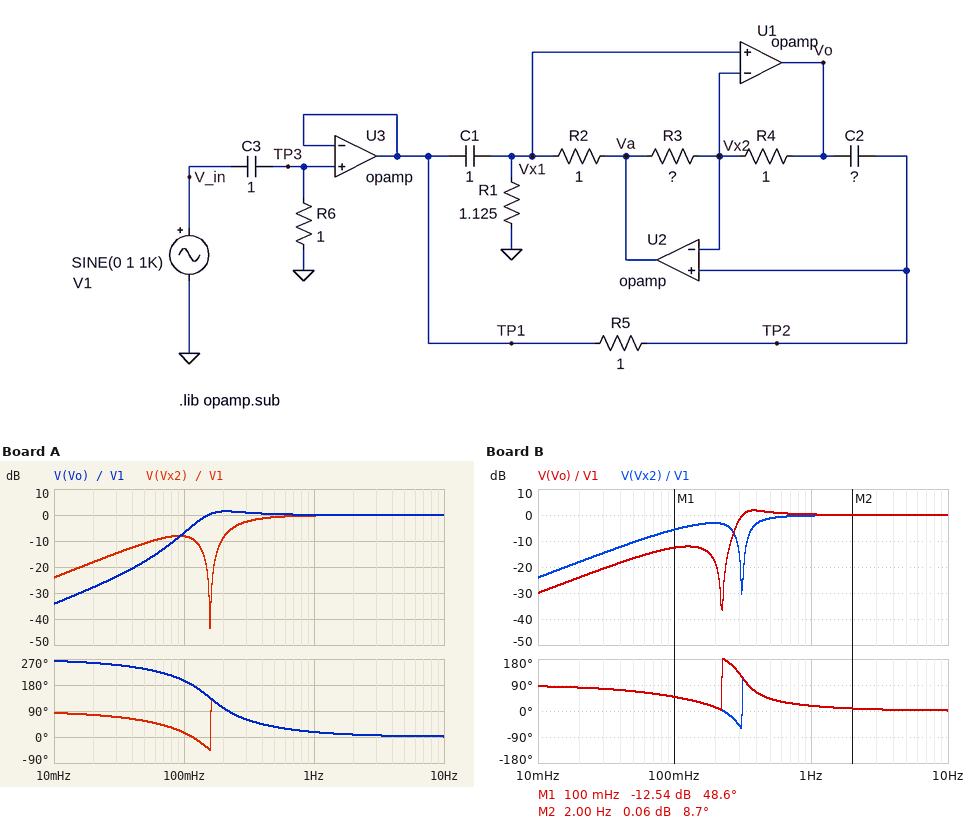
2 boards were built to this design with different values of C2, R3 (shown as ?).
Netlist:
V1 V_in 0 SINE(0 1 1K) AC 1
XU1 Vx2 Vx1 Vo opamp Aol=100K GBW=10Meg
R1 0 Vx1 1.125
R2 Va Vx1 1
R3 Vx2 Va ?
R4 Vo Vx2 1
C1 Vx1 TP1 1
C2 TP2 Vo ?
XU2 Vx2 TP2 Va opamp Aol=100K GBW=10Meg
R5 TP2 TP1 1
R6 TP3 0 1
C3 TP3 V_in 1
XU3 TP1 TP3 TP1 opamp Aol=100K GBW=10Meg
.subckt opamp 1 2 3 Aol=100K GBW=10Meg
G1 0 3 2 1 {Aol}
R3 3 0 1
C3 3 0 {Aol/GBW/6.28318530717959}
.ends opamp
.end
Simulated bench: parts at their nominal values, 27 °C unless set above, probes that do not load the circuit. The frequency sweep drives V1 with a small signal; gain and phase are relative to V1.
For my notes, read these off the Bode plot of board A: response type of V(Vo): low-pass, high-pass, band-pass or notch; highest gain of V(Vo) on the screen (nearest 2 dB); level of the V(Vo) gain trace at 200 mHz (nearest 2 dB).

high-pass
2 dB
2 dB
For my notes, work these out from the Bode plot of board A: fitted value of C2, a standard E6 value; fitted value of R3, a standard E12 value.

680 mF
0.68 Ω
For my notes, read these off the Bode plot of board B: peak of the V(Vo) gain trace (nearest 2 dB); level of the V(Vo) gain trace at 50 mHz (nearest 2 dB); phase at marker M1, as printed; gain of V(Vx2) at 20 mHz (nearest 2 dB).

2 dB
-16 dB
48.6 deg
-18 dB
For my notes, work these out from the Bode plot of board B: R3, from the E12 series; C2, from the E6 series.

1.8 Ω
470 mF
